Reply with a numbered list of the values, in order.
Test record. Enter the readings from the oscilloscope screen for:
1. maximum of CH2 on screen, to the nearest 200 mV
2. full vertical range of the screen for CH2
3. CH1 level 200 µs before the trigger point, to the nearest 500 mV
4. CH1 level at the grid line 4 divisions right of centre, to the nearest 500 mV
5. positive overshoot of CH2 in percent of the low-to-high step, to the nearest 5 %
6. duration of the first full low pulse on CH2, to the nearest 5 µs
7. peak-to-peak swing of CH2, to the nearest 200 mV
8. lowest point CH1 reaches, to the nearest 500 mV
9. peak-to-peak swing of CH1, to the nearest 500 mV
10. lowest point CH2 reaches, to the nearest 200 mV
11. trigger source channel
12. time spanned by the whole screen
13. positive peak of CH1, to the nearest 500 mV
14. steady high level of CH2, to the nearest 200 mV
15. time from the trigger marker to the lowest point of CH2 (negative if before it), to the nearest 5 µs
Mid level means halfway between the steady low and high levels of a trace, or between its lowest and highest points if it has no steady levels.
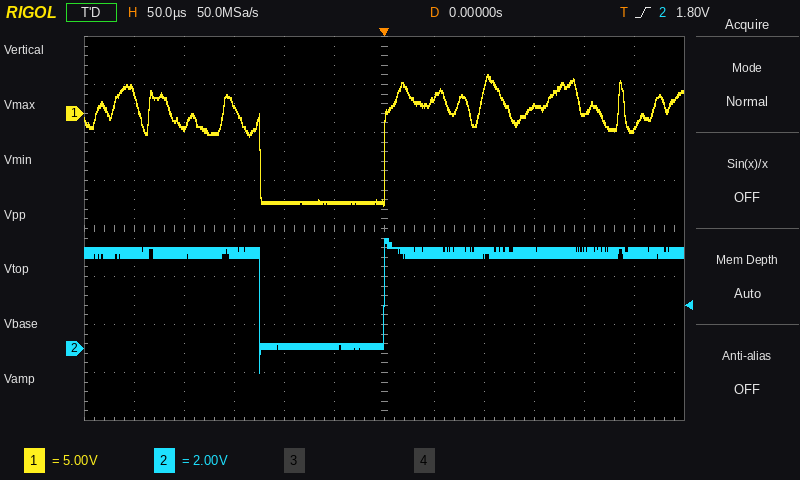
1. 4.6 V
2. 16 V
3. -1.5 V
4. 0.0 V
5. 15 %
6. 125 µs
7. 5.6 V
8. -9.5 V
9. 13.5 V
10. -1.0 V
11. CH2
12. 600 µs
13. 4.0 V
14. 4.0 V
15. -125 µs
